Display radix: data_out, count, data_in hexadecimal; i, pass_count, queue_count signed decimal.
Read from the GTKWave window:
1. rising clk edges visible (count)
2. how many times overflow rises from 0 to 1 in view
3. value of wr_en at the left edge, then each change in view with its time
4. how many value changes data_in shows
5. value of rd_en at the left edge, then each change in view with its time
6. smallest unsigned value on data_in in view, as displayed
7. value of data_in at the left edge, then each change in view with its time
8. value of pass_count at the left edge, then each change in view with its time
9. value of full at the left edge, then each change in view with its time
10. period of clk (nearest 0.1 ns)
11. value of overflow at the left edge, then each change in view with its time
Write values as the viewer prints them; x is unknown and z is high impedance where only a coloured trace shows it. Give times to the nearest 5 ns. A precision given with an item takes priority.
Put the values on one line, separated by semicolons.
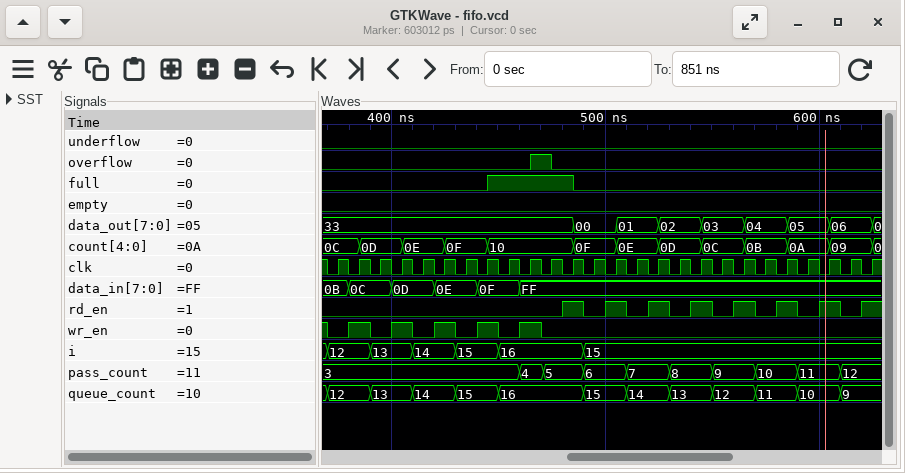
26; 1; 1, 0 at 370 ns, 1 at 380 ns, 0 at 390 ns, 1 at 400 ns, 0 at 410 ns, 1 at 420 ns, 0 at 430 ns, 1 at 440 ns, 0 at 450 ns, 1 at 460 ns, 0 at 470 ns; 5; 0, 1 at 480 ns, 0 at 490 ns, 1 at 500 ns, 0 at 510 ns, 1 at 520 ns, 0 at 530 ns, 1 at 540 ns, 0 at 550 ns, 1 at 560 ns, 0 at 570 ns, 1 at 580 ns, 0 at 590 ns, 1 at 600 ns, 0 at 610 ns, 1 at 620 ns; 0B; 0B, 0C at 380 ns, 0D at 400 ns, 0E at 420 ns, 0F at 440 ns, FF at 460 ns; 3, 4 at 460 ns, 5 at 470 ns, 6 at 490 ns, 7 at 510 ns, 8 at 530 ns, 9 at 550 ns, 10 at 570 ns, 11 at 590 ns, 12 at 610 ns; 0, 1 at 445 ns, 0 at 485 ns; 10 ns; 0, 1 at 465 ns, 0 at 475 ns
